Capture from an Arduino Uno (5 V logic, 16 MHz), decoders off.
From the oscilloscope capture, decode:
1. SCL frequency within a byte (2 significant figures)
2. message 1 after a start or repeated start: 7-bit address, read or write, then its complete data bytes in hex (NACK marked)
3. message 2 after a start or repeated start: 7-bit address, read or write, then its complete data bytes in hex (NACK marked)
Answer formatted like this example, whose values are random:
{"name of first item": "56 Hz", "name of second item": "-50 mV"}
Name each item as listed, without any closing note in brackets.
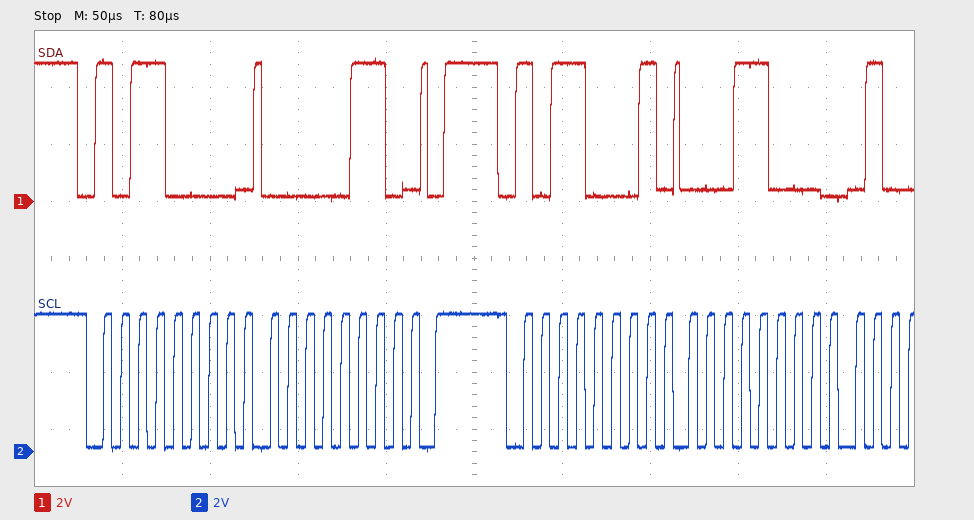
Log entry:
{"SCL frequency within a byte": "100 kHz", "message 1 after a start or repeated start: 7-bit address, read or write, then its complete data bytes in hex": "0x58 write: 06", "message 2 after a start or repeated start: 7-bit address, read or write, then its complete data bytes in hex": "0x58 read: 18"}
